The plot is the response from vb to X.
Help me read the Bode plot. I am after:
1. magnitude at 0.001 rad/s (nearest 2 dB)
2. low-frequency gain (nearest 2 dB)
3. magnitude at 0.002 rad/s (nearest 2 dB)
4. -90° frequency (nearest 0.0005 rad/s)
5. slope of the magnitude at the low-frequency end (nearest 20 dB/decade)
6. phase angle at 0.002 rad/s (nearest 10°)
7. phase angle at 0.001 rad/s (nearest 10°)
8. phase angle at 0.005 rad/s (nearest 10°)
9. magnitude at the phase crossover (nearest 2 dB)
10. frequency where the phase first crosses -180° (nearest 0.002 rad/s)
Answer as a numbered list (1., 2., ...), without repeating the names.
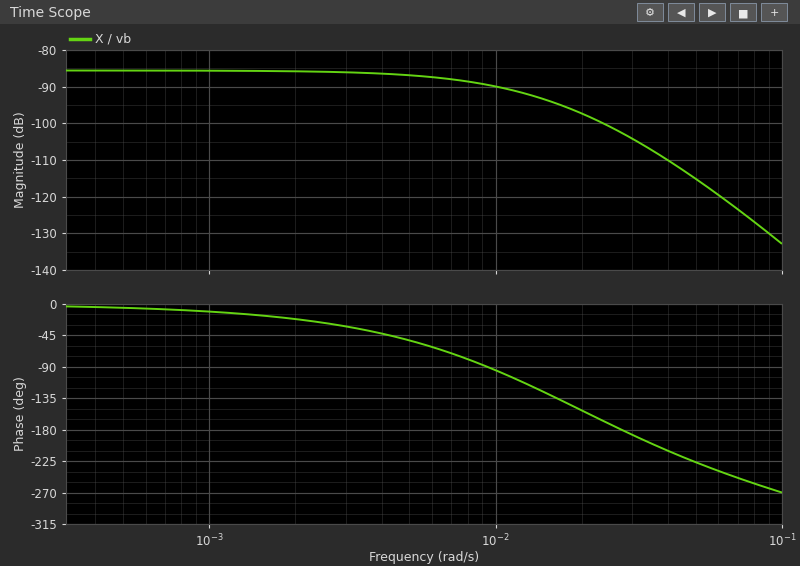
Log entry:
1. -86 dB
2. -86 dB
3. -86 dB
4. 0.0095 rad/s
5. 0 dB/decade
6. -20°
7. -10°
8. -50°
9. -102 dB
10. 0.028 rad/s
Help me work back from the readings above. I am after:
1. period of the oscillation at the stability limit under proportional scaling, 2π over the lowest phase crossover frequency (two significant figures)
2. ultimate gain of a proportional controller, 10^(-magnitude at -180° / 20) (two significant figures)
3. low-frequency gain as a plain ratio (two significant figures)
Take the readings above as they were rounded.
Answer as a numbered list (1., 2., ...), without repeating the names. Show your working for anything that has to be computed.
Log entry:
1. 2π / 0.028 = 220 s
2. 10^(102 / 20) = 130000
3. 10^(-86 / 20) = 0.000050
